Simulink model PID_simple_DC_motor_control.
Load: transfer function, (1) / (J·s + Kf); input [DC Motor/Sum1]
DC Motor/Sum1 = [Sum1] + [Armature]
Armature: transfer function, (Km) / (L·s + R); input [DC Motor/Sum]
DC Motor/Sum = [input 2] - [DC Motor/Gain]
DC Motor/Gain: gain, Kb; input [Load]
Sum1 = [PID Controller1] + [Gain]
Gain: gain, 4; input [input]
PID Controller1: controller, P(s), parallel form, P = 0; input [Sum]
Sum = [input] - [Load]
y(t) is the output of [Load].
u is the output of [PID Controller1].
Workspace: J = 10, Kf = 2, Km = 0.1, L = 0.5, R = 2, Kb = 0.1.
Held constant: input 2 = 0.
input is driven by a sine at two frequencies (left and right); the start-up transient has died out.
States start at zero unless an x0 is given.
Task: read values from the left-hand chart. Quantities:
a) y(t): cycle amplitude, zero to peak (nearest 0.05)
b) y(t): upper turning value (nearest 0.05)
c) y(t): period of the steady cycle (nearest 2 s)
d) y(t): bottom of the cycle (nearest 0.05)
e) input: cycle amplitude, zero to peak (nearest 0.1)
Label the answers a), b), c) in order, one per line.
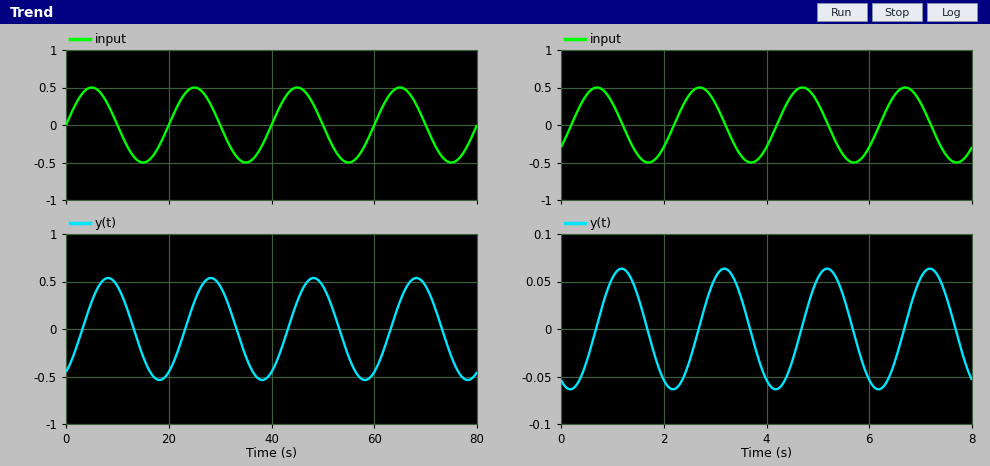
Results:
a) 0.55
b) 0.55
c) 20 s
d) -0.55
e) 0.5
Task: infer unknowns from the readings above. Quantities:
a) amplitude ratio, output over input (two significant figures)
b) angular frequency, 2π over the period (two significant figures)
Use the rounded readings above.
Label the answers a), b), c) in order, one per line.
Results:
a) 1.1
b) 0.31 rad/s
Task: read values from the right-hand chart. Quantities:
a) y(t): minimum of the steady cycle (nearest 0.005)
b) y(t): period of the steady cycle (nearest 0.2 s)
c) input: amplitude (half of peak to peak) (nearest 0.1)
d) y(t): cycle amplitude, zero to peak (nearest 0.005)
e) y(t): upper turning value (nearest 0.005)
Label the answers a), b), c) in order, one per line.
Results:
a) -0.065
b) 2.0 s
c) 0.5
d) 0.065
e) 0.065
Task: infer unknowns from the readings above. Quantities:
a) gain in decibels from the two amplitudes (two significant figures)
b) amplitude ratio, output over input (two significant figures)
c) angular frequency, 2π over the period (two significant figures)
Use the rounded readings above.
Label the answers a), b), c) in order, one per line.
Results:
a) -18 dB
b) 0.13
c) 3.1 rad/s
